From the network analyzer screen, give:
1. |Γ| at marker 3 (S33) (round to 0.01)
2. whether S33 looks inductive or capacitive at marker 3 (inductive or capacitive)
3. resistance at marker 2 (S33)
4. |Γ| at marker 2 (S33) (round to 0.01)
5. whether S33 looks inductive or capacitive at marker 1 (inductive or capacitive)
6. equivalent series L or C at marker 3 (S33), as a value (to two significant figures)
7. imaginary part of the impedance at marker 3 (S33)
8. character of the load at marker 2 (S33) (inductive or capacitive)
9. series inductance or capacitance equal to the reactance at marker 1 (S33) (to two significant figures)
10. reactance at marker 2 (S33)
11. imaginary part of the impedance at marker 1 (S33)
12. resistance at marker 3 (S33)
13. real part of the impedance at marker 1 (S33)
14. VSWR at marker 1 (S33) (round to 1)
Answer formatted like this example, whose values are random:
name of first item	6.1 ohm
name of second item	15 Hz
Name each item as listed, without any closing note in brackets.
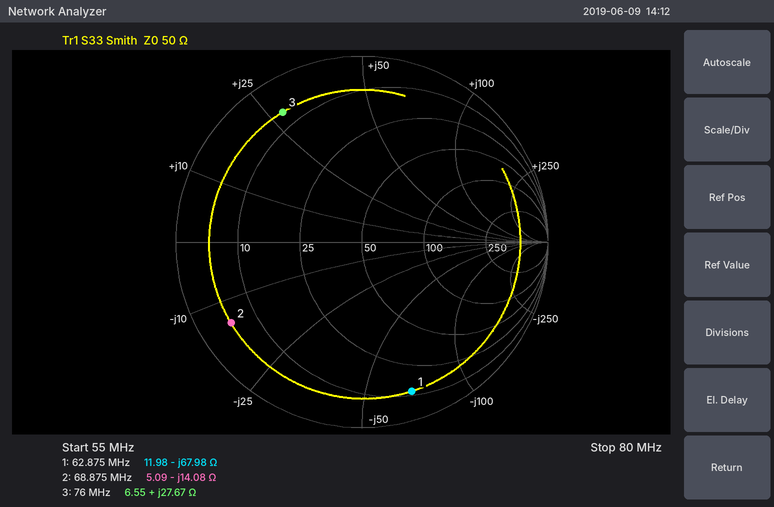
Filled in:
|Γ| at marker 3 (S33)	0.82
whether S33 looks inductive or capacitive at marker 3	inductive
resistance at marker 2	5.09 Ω
|Γ| at marker 2 (S33)	0.83
whether S33 looks inductive or capacitive at marker 1	capacitive
equivalent series L or C at marker 3 (S33), as a value	58 nH
imaginary part of the impedance at marker 3	+27.67 Ω
character of the load at marker 2 (S33)	capacitive
series inductance or capacitance equal to the reactance at marker 1 (S33)	37 pF
reactance at marker 2	-14.08 Ω
imaginary part of the impedance at marker 1	-67.98 Ω
resistance at marker 3	6.55 Ω
real part of the impedance at marker 1	11.98 Ω
VSWR at marker 1 (S33)	12
